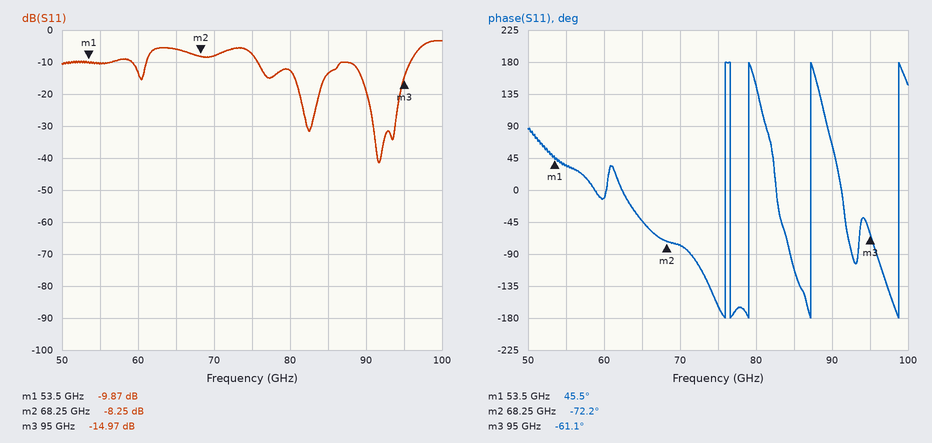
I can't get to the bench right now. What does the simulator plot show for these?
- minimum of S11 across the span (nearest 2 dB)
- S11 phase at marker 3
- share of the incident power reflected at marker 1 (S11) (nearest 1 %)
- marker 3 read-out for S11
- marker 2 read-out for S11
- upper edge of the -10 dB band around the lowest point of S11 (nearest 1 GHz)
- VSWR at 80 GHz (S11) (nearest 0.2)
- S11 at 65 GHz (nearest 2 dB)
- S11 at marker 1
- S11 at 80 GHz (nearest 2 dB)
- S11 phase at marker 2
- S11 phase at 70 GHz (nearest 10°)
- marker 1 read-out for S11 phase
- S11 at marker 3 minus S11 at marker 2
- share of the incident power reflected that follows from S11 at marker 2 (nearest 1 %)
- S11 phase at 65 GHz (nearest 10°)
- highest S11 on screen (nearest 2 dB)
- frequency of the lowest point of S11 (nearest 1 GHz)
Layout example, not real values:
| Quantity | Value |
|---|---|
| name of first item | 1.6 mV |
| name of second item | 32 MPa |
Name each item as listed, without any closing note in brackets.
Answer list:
| Quantity | Value |
|---|---|
| minimum of S11 across the span | -42 dB |
| S11 phase at marker 3 | -61.1° |
| share of the incident power reflected at marker 1 (S11) | 10 % |
| marker 3 read-out for S11 | -14.97 dB |
| marker 2 read-out for S11 | -8.25 dB |
| upper edge of the -10 dB band around the lowest point of S11 | 96 GHz |
| VSWR at 80 GHz (S11) | 1.6 |
| S11 at 65 GHz | -6 dB |
| S11 at marker 1 | -9.87 dB |
| S11 at 80 GHz | -12 dB |
| S11 phase at marker 2 | -72.2° |
| S11 phase at 70 GHz | -80° |
| marker 1 read-out for S11 phase | 45.5° |
| S11 at marker 3 minus S11 at marker 2 | -6.72 dB |
| share of the incident power reflected that follows from S11 at marker 2 | 15 % |
| S11 phase at 65 GHz | -40° |
| highest S11 on screen | -4 dB |
| frequency of the lowest point of S11 | 92 GHz |
